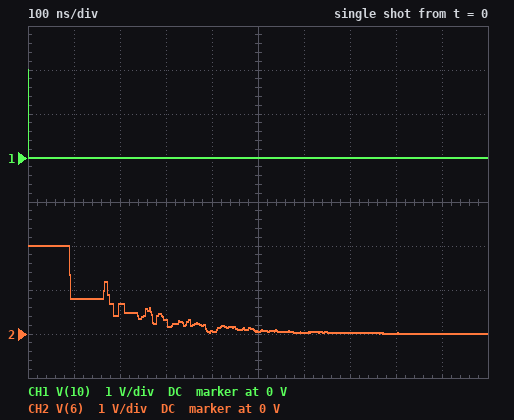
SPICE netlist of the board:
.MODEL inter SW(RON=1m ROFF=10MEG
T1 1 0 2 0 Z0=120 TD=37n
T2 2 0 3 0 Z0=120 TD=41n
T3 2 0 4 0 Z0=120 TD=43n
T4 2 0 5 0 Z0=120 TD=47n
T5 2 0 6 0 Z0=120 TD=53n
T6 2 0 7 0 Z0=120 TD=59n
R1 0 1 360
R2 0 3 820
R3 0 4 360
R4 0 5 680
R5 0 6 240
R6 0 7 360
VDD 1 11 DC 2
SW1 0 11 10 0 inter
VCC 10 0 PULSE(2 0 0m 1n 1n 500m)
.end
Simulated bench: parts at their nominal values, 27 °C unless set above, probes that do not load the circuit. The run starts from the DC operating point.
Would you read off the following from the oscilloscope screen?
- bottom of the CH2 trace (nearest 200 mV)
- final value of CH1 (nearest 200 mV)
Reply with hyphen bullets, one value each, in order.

- 0 V
- 0 V
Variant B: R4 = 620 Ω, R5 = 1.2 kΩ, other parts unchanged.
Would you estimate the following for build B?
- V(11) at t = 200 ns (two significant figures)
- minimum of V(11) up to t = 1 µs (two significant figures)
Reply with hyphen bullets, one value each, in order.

- -1.9 V
- -2.2 V
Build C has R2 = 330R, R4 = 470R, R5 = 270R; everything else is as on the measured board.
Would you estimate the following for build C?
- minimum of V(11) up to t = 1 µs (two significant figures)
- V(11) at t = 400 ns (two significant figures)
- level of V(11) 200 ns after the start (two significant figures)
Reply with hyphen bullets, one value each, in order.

- -3.1 V
- -1.9 V
- -2.3 V
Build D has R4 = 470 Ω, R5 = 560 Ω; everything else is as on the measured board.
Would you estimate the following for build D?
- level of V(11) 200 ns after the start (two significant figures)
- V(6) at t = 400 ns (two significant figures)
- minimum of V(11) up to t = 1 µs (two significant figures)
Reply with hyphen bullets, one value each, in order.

- -2.0 V
- 74 mV
- -2.4 V
